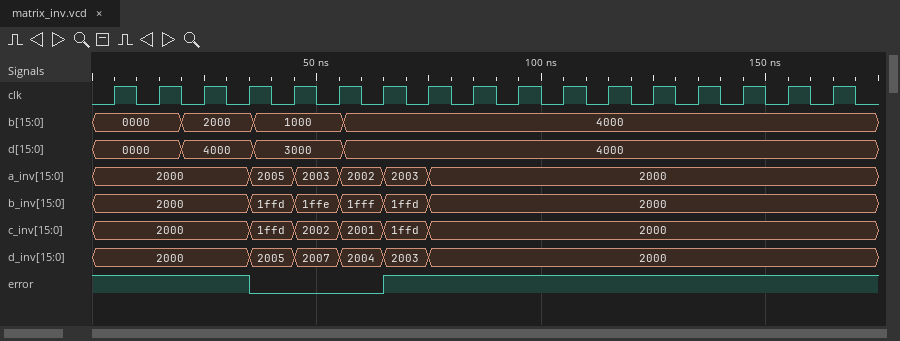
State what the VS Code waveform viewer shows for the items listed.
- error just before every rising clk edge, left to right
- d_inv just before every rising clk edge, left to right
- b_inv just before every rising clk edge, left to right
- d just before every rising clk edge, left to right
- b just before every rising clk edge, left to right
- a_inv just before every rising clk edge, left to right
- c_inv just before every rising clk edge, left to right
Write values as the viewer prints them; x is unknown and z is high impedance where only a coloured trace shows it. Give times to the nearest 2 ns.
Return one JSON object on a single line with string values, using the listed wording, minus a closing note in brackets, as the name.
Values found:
{"error just before every rising clk edge, left to right": "1 1 1 1 0 0 0 1 1 1 1 1 1 1 1 1 1", "d_inv just before every rising clk edge, left to right": "2000, 2000, 2000, 2000, 2005, 2007, 2004, 2003, 2000, 2000, 2000, 2000, 2000, 2000, 2000, 2000, 2000", "b_inv just before every rising clk edge, left to right": "2000, 2000, 2000, 2000, 1ffd, 1ffe, 1fff, 1ffd, 2000, 2000, 2000, 2000, 2000, 2000, 2000, 2000, 2000", "d just before every rising clk edge, left to right": "0000, 0000, 4000, 4000, 3000, 3000, 4000, 4000, 4000, 4000, 4000, 4000, 4000, 4000, 4000, 4000, 4000", "b just before every rising clk edge, left to right": "0000, 0000, 2000, 2000, 1000, 1000, 4000, 4000, 4000, 4000, 4000, 4000, 4000, 4000, 4000, 4000, 4000", "a_inv just before every rising clk edge, left to right": "2000, 2000, 2000, 2000, 2005, 2003, 2002, 2003, 2000, 2000, 2000, 2000, 2000, 2000, 2000, 2000, 2000", "c_inv just before every rising clk edge, left to right": "2000, 2000, 2000, 2000, 1ffd, 2002, 2001, 1ffd, 2000, 2000, 2000, 2000, 2000, 2000, 2000, 2000, 2000"}
